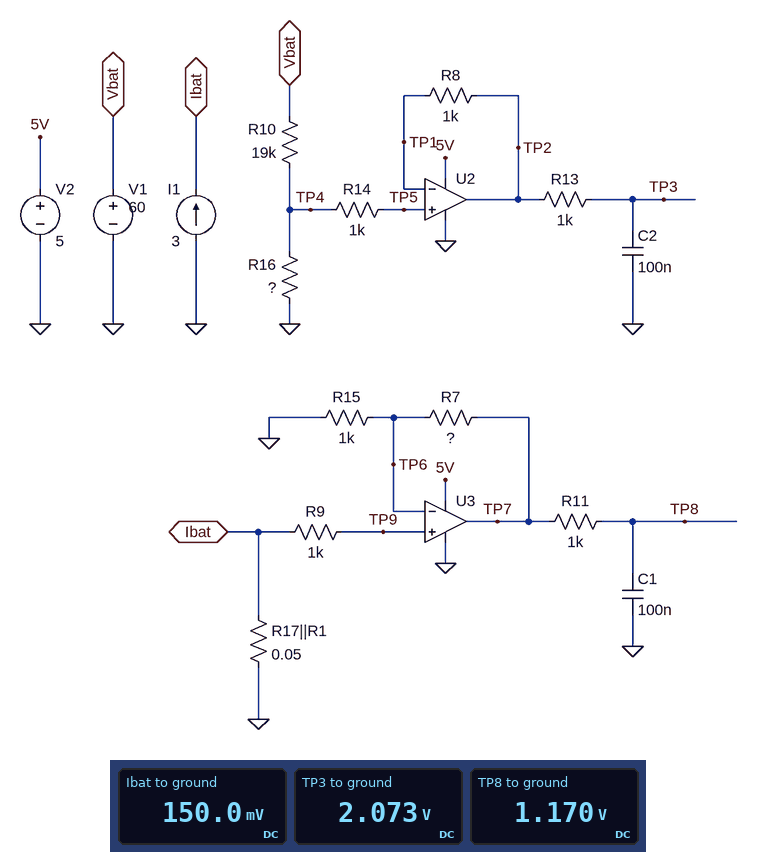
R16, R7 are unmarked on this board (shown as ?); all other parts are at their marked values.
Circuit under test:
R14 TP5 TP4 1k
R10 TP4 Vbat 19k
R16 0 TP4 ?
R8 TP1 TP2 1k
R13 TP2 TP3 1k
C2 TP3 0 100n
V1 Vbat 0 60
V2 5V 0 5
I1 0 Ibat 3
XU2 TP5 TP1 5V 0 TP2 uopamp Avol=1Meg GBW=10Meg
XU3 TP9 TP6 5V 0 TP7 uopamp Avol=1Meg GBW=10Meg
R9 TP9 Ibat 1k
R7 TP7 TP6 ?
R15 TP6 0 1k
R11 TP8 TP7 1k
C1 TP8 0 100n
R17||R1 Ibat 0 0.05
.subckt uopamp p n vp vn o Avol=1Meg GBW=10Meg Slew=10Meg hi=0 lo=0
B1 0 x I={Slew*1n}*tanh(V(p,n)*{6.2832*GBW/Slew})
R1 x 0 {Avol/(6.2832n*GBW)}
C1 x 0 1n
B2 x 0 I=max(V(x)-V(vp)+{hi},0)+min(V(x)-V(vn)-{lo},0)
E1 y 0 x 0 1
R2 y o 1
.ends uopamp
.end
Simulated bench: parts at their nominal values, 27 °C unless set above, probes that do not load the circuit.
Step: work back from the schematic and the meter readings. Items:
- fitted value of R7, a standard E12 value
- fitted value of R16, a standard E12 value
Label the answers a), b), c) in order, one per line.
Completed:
a) 6.8 kΩ
b) 680 Ω
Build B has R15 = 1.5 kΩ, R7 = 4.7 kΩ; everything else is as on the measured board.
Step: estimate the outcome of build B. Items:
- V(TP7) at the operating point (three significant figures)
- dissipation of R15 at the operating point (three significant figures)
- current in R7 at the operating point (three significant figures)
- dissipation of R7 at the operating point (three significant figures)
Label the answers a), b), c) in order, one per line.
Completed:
a) 620 mV
b) 15.0 µW
c) 100 µA
d) 47.0 µW
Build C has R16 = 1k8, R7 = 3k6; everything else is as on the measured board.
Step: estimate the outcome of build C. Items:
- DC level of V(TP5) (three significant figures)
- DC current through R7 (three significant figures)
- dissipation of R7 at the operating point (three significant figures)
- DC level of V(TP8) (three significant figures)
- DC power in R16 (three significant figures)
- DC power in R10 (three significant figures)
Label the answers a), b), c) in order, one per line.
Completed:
a) 5.19 V
b) 150 µA
c) 81.0 µW
d) 690 mV
e) 15.0 mW
f) 158 mW
